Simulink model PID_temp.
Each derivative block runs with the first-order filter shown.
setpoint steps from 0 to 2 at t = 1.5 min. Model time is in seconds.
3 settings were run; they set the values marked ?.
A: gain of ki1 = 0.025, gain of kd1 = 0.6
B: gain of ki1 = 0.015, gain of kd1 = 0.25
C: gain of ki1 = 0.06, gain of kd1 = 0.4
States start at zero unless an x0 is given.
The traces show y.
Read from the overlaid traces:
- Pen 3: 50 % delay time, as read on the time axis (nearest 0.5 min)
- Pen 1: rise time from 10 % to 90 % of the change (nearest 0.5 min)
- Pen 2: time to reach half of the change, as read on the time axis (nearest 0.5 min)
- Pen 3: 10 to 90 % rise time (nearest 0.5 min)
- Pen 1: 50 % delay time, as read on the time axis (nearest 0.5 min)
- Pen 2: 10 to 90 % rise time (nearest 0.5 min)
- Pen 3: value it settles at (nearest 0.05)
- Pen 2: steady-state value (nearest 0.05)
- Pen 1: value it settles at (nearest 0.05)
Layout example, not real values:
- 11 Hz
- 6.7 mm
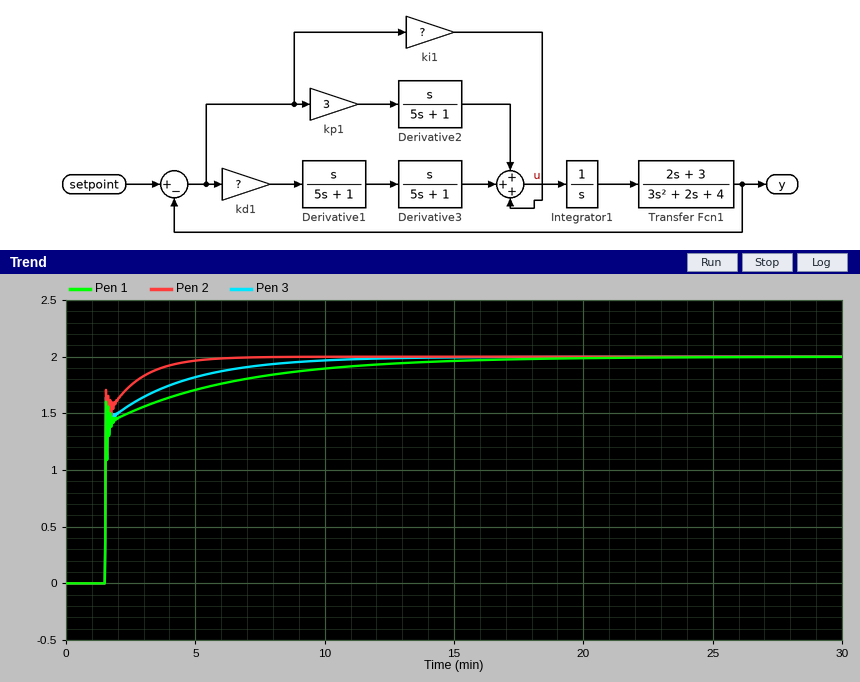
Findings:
- 1.5 min
- 5.5 min
- 1.5 min
- 3.0 min
- 1.5 min
- 1.5 min
- 2.00
- 2.00
- 2.00
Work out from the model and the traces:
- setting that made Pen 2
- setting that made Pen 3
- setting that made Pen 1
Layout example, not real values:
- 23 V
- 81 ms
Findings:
- C
- A
- B
